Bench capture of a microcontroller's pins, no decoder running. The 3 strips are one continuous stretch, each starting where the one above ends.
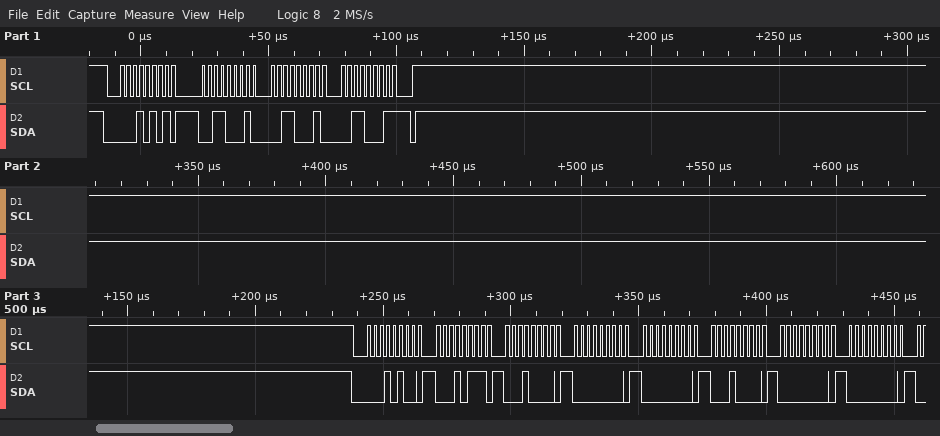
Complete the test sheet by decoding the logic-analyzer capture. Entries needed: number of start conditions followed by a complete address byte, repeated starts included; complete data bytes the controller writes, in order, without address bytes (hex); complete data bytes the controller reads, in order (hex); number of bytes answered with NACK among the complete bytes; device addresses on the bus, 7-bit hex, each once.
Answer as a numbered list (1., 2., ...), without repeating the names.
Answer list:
1. 2
2. 17 10 00 00 10 00 00
3. 31 31 31
4. 1
5. 0x0A
